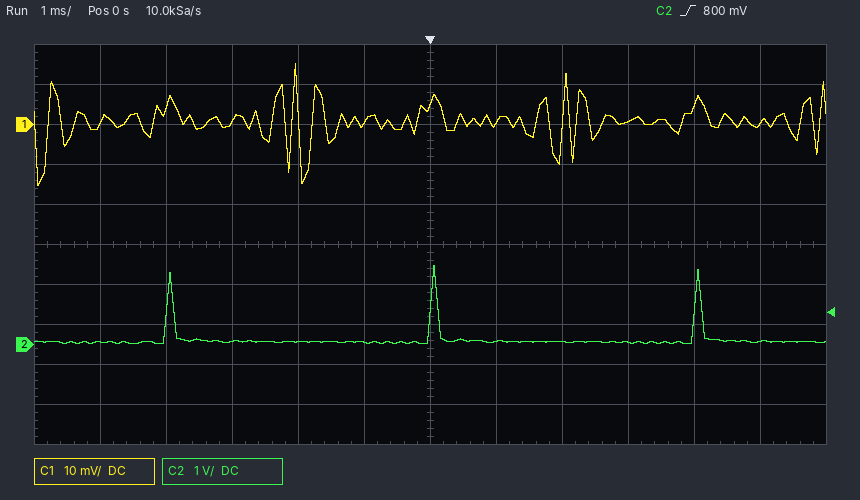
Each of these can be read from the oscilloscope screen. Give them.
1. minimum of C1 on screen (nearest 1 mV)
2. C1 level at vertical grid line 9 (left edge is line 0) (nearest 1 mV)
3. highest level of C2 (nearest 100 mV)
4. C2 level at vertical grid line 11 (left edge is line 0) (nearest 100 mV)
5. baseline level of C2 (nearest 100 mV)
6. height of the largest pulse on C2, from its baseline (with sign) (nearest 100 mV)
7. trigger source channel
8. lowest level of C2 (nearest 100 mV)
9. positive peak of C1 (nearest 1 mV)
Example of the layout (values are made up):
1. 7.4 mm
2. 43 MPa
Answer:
1. -15 mV
2. 1 mV
3. 2.0 V
4. 100 mV
5. 100 mV
6. +1.9 V
7. C2
8. 0.0 V
9. 15 mV
